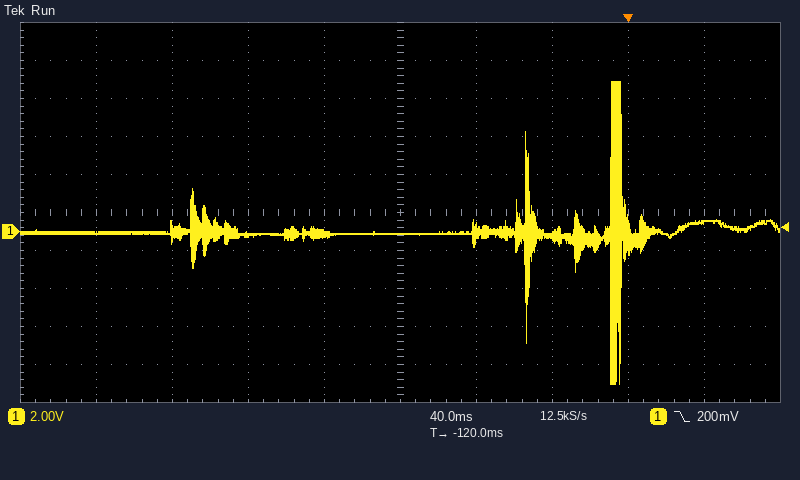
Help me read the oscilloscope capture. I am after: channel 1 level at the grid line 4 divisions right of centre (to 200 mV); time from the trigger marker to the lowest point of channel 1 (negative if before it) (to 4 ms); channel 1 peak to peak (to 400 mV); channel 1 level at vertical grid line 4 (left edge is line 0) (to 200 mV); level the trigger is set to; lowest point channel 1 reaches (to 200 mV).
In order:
400 mV
-8 ms
16.0 V
-200 mV
200 mV
-8.0 V
